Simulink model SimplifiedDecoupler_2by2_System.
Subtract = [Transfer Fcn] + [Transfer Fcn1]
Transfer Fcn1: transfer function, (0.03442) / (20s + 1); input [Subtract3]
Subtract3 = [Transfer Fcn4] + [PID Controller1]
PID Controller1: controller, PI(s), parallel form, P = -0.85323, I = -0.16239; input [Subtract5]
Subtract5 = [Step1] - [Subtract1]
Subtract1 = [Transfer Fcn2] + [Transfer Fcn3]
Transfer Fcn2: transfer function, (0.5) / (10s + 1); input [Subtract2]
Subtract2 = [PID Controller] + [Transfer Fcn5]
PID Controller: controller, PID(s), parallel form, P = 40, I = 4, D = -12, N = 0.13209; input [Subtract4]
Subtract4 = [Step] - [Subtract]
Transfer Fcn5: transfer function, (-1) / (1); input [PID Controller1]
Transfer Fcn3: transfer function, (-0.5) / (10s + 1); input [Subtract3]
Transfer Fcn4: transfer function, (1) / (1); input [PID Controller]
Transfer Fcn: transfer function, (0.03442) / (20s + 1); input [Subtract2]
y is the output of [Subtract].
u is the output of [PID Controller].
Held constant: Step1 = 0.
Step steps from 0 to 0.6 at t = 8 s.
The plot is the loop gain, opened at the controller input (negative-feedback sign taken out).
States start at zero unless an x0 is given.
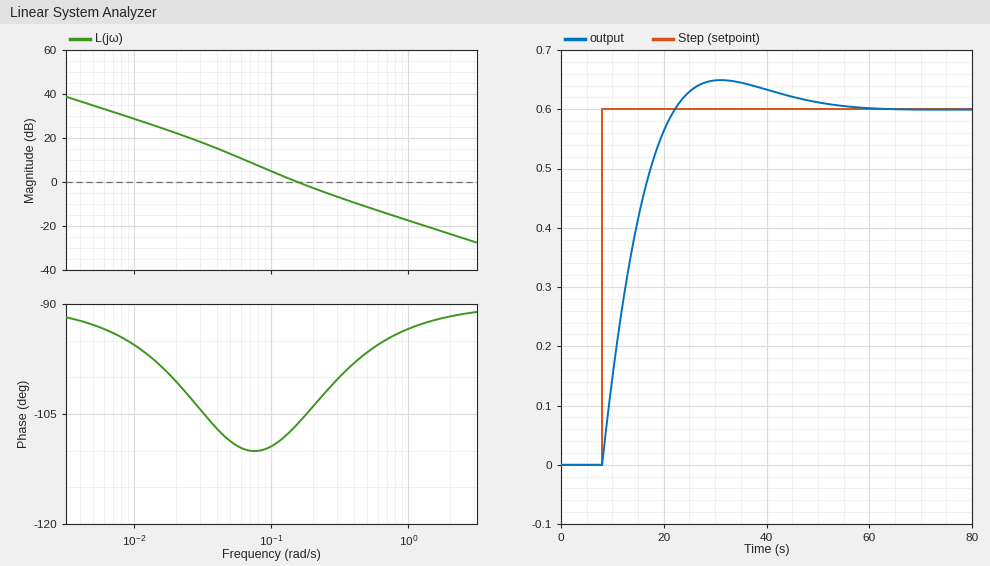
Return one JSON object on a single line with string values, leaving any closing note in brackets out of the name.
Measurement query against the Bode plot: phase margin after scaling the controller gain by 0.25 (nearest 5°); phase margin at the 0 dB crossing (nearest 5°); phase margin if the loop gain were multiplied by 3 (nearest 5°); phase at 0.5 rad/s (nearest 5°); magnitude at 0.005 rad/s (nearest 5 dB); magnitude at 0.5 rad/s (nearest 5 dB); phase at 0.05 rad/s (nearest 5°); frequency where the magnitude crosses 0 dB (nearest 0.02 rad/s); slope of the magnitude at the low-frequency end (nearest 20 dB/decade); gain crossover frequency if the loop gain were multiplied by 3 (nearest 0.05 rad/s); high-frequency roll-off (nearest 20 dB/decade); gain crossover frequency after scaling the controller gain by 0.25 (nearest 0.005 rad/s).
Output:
{"phase margin after scaling the controller gain by 0.25": "70°", "phase margin at the 0 dB crossing": "75°", "phase margin if the loop gain were multiplied by 3": "80°", "phase at 0.5 rad/s": "-95°", "magnitude at 0.005 rad/s": "35 dB", "magnitude at 0.5 rad/s": "-10 dB", "phase at 0.05 rad/s": "-110°", "frequency where the magnitude crosses 0 dB": "0.16 rad/s", "slope of the magnitude at the low-frequency end": "-20 dB/decade", "gain crossover frequency if the loop gain were multiplied by 3": "0.40 rad/s", "high-frequency roll-off": "-20 dB/decade", "gain crossover frequency after scaling the controller gain by 0.25": "0.055 rad/s"}
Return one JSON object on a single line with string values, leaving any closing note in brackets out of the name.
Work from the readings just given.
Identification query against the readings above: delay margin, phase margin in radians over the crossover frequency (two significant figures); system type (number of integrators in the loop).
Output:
{"delay margin, phase margin in radians over the crossover frequency": "8.2 s", "system type": "1"}
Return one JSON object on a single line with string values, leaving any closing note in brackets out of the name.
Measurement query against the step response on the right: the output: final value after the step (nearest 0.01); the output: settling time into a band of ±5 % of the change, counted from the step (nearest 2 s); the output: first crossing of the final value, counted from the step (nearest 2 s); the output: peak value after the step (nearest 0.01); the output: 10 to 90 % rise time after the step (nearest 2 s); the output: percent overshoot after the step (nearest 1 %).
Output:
{"the output: final value after the step": "0.60", "the output: settling time into a band of ±5 % of the change, counted from the step": "34 s", "the output: first crossing of the final value, counted from the step": "14 s", "the output: peak value after the step": "0.65", "the output: 10 to 90 % rise time after the step": "10 s", "the output: percent overshoot after the step": "8 %"}
